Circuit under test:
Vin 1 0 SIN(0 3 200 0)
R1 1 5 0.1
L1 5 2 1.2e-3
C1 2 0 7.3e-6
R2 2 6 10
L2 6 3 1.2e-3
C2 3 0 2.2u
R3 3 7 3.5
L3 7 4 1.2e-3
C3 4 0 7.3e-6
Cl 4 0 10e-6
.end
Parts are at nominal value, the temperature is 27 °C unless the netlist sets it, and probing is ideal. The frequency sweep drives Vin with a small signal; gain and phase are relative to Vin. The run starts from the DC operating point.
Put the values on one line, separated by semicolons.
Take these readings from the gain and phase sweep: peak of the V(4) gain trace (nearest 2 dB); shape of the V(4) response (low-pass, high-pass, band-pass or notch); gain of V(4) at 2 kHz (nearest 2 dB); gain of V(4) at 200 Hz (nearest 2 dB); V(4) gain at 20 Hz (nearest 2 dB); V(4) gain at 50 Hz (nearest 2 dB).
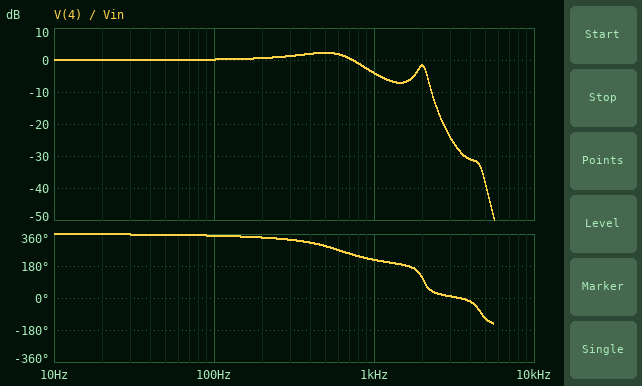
2 dB; low-pass; -2 dB; 0 dB; 0 dB; 0 dB
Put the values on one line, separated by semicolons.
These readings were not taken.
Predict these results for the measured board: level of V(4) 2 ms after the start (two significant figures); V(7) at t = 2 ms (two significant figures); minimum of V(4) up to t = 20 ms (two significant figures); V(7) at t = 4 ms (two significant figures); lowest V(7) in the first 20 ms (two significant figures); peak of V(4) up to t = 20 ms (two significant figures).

2.7 V; 2.6 V; -3.2 V; -3.1 V; -3.1 V; 3.3 V
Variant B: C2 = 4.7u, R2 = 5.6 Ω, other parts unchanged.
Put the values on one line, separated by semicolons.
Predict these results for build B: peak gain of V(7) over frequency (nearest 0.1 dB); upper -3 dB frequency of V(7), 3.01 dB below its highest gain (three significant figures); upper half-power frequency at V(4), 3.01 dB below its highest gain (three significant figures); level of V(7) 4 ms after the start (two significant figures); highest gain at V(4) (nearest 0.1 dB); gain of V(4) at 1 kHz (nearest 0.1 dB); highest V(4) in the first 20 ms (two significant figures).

7.9 dB; 2.11 kHz; 727 Hz; -3.2 V; 5.4 dB; -3.2 dB; 3.6 V
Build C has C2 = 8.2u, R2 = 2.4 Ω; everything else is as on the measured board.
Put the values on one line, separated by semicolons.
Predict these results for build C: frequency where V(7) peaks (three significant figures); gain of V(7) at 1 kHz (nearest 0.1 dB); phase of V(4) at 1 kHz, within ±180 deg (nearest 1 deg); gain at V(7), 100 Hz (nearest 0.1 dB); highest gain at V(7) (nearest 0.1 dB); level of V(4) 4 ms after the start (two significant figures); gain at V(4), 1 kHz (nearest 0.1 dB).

536 Hz; -17.8 dB; -172 deg; 0.2 dB; 7.4 dB; -3.5 V; -2.9 dB
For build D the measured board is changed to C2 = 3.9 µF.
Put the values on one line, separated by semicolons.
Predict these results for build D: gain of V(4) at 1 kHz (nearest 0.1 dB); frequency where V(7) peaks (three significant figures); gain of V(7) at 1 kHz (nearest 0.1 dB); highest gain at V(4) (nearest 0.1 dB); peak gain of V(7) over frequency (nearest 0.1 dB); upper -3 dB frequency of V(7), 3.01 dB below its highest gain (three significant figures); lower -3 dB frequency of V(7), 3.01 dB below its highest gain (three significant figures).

-4.2 dB; 1.99 kHz; -19.1 dB; 2.1 dB; 6.6 dB; 2.14 kHz; 1.86 kHz
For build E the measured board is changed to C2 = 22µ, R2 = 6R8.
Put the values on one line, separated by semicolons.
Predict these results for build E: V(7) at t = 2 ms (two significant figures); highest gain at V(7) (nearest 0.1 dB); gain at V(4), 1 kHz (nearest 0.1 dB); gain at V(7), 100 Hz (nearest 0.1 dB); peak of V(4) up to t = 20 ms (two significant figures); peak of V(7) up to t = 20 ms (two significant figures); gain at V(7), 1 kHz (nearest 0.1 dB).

3.0 V; 1.6 dB; -5.1 dB; 0.2 dB; 3.4 V; 3.3 V; -20.0 dB
